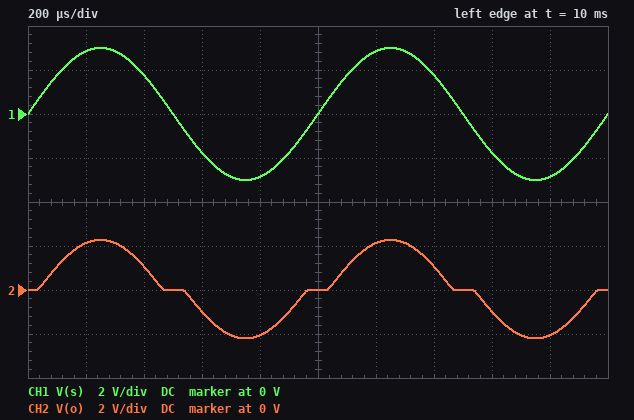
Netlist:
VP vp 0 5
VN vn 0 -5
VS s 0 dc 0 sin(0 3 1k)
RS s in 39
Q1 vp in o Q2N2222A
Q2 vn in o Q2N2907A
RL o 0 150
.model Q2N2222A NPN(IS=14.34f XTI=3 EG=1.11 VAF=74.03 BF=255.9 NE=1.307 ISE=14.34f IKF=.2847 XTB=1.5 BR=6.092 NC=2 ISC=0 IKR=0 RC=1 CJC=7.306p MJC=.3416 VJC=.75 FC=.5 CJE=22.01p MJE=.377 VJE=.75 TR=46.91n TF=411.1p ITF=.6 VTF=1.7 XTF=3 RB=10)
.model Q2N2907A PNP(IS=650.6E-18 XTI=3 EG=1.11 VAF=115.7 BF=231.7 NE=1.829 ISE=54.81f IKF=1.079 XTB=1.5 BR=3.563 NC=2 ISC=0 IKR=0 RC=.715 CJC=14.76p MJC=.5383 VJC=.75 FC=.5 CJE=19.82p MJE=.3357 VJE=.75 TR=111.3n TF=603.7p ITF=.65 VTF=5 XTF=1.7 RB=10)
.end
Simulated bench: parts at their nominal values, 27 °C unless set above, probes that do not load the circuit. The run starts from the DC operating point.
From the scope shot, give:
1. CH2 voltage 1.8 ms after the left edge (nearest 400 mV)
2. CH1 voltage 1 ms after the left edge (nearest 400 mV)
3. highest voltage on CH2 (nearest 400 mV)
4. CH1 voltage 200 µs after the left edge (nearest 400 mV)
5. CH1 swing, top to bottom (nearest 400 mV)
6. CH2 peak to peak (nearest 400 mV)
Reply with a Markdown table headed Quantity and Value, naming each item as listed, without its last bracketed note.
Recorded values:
| Quantity | Value |
|---|---|
| CH2 voltage 1.8 ms after the left edge | -2.0 V |
| CH1 voltage 1 ms after the left edge | 0 V |
| highest voltage on CH2 | 2.4 V |
| CH1 voltage 200 µs after the left edge | 2.8 V |
| CH1 swing, top to bottom | 6.0 V |
| CH2 peak to peak | 4.4 V |
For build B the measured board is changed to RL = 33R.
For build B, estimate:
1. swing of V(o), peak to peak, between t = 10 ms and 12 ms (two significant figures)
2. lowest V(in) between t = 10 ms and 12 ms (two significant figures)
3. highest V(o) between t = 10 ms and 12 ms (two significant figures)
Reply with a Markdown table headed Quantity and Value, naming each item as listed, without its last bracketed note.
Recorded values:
| Quantity | Value |
|---|---|
| swing of V(o), peak to peak, between t = 10 ms and 12 ms | 4.4 V |
| lowest V(in) between t = 10 ms and 12 ms | -3.0 V |
| highest V(o) between t = 10 ms and 12 ms | 2.2 V |
